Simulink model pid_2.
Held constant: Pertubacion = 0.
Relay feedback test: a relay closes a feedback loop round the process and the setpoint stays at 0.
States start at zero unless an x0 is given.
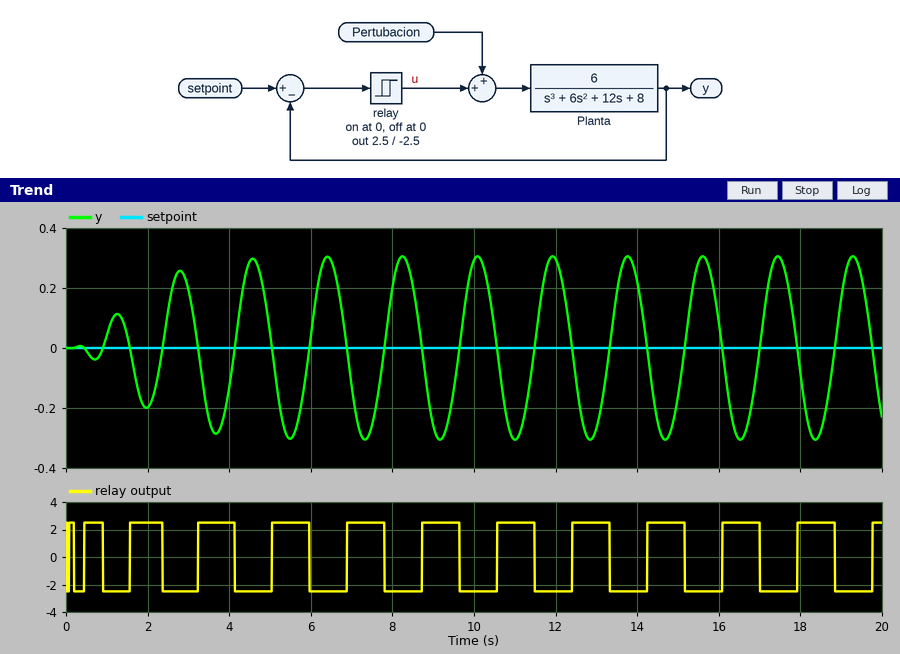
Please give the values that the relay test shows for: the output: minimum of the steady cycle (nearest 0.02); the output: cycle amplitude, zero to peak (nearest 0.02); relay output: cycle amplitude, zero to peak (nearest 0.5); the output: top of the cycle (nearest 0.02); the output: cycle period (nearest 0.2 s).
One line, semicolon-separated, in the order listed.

-0.30; 0.30; 2.5; 0.30; 1.8 s
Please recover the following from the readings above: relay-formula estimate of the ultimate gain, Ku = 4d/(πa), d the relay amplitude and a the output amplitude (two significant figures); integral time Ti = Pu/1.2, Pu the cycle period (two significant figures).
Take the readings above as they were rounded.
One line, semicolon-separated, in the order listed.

11; 1.5 s
